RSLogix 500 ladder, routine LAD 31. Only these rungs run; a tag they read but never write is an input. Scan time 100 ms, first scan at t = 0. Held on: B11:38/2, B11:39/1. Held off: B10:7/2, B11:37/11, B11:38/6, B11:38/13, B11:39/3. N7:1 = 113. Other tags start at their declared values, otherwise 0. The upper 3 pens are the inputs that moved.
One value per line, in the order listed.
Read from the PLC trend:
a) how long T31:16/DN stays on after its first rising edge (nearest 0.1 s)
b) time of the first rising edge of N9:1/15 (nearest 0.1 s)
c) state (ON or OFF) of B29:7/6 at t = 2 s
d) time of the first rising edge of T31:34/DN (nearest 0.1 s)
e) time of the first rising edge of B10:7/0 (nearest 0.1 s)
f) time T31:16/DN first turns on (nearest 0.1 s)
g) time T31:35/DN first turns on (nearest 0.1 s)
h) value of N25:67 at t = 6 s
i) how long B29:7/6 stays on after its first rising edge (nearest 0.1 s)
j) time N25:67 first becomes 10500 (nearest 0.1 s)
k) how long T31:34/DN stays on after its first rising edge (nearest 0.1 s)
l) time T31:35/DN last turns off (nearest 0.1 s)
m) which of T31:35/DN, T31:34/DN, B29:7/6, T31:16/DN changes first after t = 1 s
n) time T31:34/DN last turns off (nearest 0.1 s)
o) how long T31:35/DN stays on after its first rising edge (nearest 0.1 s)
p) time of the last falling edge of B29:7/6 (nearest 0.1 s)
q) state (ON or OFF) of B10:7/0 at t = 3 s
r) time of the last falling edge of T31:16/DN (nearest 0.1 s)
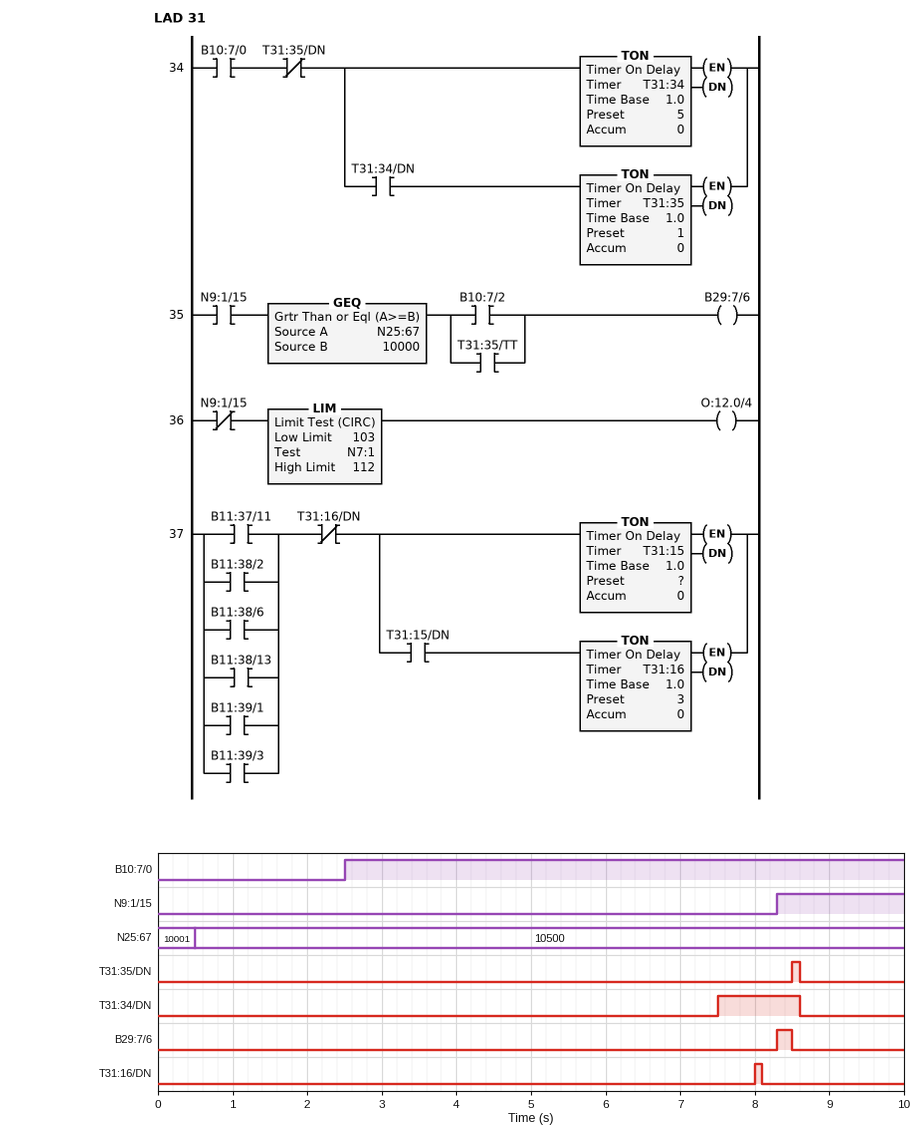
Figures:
0.1 s
8.3 s
OFF
7.5 s
2.5 s
8.0 s
8.5 s
10500
0.2 s
0.5 s
1.1 s
8.6 s
T31:34/DN
8.6 s
0.1 s
8.5 s
ON
8.1 s
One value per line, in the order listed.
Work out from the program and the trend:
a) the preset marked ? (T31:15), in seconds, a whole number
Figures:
5 s
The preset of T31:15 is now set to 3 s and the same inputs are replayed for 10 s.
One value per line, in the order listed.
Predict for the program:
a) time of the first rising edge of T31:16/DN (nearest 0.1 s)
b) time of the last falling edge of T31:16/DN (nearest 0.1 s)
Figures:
6.0 s
6.1 s
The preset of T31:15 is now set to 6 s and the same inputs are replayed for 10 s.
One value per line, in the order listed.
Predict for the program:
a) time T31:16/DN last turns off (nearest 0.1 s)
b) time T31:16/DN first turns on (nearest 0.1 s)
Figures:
9.1 s
9.0 s
